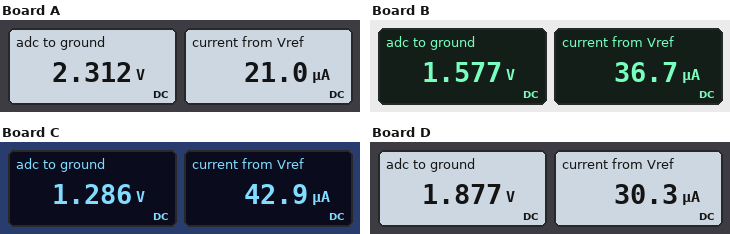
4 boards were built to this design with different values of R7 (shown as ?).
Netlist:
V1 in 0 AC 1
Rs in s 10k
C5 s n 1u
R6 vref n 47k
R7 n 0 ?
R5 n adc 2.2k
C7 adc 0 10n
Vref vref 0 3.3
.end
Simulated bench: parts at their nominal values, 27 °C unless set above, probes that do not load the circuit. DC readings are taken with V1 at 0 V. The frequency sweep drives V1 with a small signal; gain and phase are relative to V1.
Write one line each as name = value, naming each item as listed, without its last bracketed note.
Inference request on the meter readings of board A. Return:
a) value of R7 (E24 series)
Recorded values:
value of R7 = 110 kΩ
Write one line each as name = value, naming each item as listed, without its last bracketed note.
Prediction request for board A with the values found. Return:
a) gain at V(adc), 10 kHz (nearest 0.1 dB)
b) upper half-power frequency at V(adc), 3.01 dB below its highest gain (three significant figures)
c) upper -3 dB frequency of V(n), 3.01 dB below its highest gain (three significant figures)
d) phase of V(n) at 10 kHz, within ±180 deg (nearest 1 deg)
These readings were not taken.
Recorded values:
gain at V(adc), 10 kHz = -18.3 dB
upper half-power frequency at V(adc), 3.01 dB below its highest gain = 1.63 kHz
upper -3 dB frequency of V(n), 3.01 dB below its highest gain = 1.72 kHz
phase of V(n) at 10 kHz, within ±180 deg = -27 deg
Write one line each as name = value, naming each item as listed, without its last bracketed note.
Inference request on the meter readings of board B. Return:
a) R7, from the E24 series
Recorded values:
R7, from the E24 series = 43 kΩ
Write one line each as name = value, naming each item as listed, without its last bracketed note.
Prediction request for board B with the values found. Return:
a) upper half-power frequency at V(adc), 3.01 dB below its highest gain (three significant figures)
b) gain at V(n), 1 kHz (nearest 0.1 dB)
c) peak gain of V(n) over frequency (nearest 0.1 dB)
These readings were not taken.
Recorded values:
upper half-power frequency at V(adc), 3.01 dB below its highest gain = 1.76 kHz
gain at V(n), 1 kHz = -4.4 dB
peak gain of V(n) over frequency = -3.3 dB
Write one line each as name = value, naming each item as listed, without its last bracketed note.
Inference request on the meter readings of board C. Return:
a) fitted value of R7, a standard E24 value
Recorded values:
fitted value of R7, a standard E24 value = 30 kΩ
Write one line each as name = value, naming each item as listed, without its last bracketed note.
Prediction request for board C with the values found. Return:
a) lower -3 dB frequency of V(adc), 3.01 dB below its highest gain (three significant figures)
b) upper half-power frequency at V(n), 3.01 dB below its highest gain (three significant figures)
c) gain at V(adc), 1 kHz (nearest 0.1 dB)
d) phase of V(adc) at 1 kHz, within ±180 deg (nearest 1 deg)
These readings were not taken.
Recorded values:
lower -3 dB frequency of V(adc), 3.01 dB below its highest gain = 5.56 Hz
upper half-power frequency at V(n), 3.01 dB below its highest gain = 1.99 kHz
gain at V(adc), 1 kHz = -4.9 dB
phase of V(adc) at 1 kHz, within ±180 deg = -28 deg
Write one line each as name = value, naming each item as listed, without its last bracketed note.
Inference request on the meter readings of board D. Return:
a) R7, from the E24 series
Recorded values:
R7, from the E24 series = 62 kΩ
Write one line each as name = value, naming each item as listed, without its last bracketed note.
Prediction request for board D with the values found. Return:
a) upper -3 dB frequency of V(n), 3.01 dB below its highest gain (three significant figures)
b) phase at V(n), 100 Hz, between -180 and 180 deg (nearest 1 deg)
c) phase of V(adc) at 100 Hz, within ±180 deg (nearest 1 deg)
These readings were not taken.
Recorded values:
upper -3 dB frequency of V(n), 3.01 dB below its highest gain = 1.80 kHz
phase at V(n), 100 Hz, between -180 and 180 deg = 0 deg
phase of V(adc) at 100 Hz, within ±180 deg = -1 deg
